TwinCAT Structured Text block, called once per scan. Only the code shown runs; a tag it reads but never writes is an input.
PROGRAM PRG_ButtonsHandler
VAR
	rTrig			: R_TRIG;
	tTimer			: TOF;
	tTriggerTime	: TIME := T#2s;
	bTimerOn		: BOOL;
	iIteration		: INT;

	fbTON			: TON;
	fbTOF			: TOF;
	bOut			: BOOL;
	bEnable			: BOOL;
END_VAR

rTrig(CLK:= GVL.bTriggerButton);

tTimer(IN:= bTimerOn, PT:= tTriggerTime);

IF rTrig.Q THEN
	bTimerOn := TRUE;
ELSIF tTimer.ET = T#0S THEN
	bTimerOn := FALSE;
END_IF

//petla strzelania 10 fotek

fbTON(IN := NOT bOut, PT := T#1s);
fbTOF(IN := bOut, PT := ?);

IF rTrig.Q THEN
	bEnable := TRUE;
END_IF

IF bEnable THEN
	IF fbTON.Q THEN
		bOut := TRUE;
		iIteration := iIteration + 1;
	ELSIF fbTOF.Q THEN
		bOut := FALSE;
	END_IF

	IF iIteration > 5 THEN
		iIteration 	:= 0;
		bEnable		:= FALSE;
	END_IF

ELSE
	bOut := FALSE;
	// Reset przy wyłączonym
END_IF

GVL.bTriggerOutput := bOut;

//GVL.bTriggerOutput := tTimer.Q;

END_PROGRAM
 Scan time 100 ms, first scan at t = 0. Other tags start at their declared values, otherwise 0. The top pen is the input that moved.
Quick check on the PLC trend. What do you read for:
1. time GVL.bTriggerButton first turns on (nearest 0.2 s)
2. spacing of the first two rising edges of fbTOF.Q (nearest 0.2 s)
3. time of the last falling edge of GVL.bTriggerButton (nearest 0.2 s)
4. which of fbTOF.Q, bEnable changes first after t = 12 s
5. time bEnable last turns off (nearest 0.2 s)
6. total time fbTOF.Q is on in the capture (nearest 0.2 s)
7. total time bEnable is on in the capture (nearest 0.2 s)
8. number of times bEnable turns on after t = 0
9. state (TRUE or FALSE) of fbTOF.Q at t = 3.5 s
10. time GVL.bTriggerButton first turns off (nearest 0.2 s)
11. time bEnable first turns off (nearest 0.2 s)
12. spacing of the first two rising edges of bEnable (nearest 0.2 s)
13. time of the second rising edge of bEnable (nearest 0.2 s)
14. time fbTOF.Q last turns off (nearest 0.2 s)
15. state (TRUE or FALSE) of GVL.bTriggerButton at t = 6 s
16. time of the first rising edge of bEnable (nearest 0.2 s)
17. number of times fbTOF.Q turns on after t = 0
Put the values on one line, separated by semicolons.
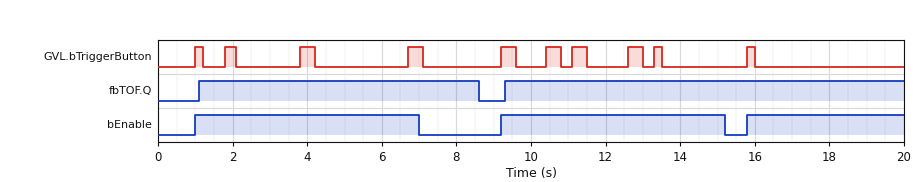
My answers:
1.0 s; 8.2 s; 16.0 s; bEnable; 15.2 s; 18.2 s; 16.2 s; 3; TRUE; 1.2 s; 7.0 s; 8.2 s; 9.2 s; 8.6 s; FALSE; 1.0 s; 2
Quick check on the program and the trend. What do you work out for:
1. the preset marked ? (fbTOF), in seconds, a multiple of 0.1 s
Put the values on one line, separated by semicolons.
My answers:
1.4 s
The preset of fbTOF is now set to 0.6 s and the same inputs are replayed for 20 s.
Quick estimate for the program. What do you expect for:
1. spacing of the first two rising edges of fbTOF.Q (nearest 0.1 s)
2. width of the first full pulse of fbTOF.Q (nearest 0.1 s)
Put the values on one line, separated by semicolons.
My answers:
1.2 s; 0.7 s
